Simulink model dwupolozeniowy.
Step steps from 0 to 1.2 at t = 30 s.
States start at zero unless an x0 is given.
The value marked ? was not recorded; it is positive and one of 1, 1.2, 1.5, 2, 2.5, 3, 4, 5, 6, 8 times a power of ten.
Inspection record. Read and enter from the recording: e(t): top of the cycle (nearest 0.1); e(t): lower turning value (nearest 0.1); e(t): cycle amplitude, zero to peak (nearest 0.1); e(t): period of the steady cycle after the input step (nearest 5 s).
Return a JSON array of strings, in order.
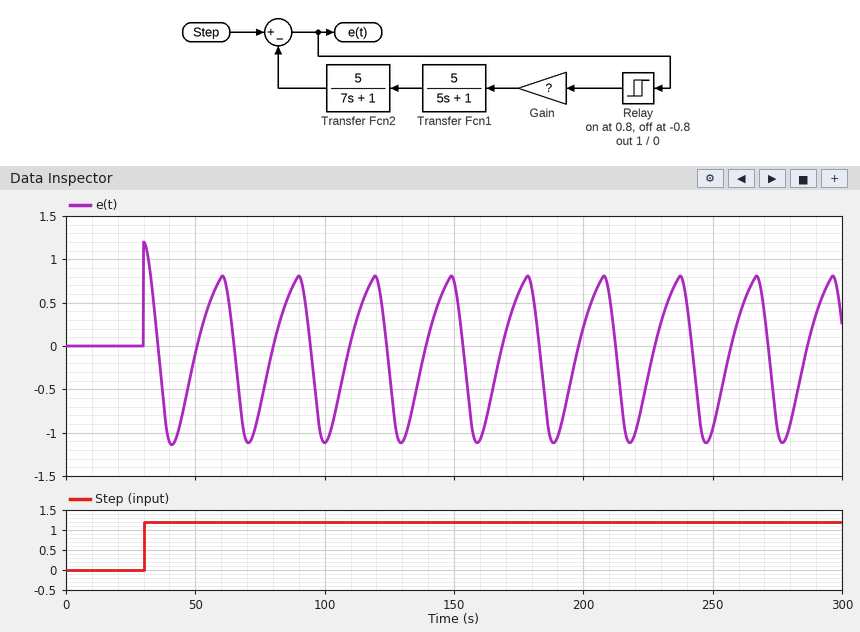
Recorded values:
["0.8", "-1.1", "1.0", "30 s"]
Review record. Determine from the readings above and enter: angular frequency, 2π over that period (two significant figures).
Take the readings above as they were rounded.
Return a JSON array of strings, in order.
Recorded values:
["0.21 rad/s"]
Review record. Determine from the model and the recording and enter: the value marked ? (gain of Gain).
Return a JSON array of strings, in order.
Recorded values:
["0.2"]
